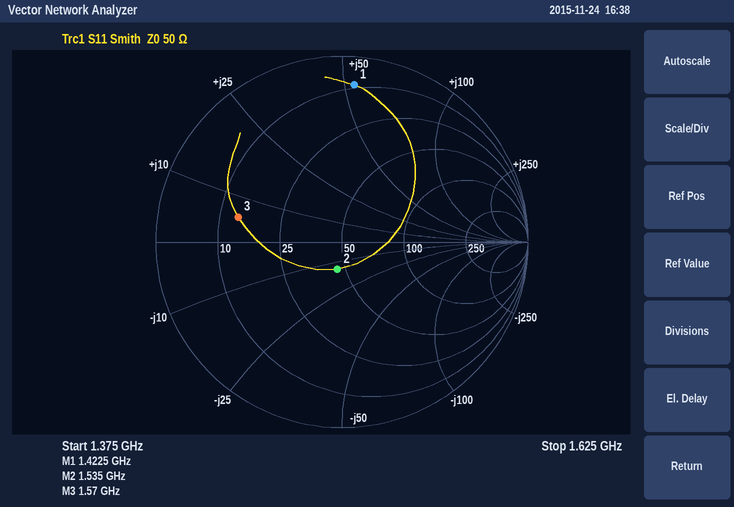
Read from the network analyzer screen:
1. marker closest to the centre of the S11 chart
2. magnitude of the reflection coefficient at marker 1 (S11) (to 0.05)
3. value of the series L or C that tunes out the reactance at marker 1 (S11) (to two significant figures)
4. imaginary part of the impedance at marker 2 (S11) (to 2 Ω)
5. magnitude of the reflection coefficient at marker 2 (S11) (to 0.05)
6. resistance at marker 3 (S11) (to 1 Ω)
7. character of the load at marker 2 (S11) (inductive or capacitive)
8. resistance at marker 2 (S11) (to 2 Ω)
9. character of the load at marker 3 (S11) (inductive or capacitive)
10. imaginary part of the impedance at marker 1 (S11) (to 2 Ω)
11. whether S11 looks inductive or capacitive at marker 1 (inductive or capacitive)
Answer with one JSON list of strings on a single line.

["marker 2", "0.85", "2.1 pF", "-14 Ω", "0.15", "14 Ω", "capacitive", "46 Ω", "inductive", "+54 Ω", "inductive"]
